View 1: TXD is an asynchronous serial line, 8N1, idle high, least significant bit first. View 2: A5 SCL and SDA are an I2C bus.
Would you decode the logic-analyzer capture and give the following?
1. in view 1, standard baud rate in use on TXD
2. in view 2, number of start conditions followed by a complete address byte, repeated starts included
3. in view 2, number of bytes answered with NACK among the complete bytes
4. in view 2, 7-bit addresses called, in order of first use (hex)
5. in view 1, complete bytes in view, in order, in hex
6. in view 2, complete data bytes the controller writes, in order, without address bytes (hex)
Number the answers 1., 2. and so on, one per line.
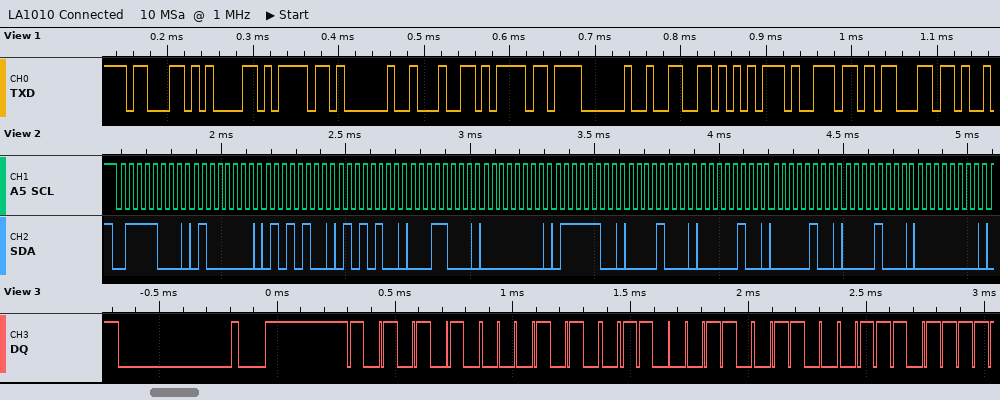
1. 115200 baud
2. 1
3. 0
4. 0x3C
5. 63 61 6F 20 64 6F 20 66 75 6E 63
6. 40 54 54 18 00 7C 08 04 04 08 00
